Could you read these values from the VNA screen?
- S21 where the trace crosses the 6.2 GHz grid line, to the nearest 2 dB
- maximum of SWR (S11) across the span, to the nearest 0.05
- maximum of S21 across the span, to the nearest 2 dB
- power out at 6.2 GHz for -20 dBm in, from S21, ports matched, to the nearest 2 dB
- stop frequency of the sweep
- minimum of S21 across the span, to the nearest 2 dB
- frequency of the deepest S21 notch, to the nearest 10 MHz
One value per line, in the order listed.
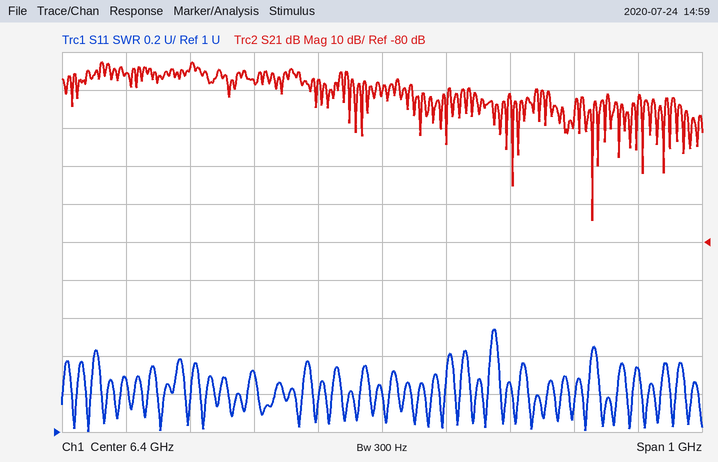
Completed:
-38 dB
1.55
-32 dB
-58 dBm
6.9 GHz
-74 dB
6.73 GHz
